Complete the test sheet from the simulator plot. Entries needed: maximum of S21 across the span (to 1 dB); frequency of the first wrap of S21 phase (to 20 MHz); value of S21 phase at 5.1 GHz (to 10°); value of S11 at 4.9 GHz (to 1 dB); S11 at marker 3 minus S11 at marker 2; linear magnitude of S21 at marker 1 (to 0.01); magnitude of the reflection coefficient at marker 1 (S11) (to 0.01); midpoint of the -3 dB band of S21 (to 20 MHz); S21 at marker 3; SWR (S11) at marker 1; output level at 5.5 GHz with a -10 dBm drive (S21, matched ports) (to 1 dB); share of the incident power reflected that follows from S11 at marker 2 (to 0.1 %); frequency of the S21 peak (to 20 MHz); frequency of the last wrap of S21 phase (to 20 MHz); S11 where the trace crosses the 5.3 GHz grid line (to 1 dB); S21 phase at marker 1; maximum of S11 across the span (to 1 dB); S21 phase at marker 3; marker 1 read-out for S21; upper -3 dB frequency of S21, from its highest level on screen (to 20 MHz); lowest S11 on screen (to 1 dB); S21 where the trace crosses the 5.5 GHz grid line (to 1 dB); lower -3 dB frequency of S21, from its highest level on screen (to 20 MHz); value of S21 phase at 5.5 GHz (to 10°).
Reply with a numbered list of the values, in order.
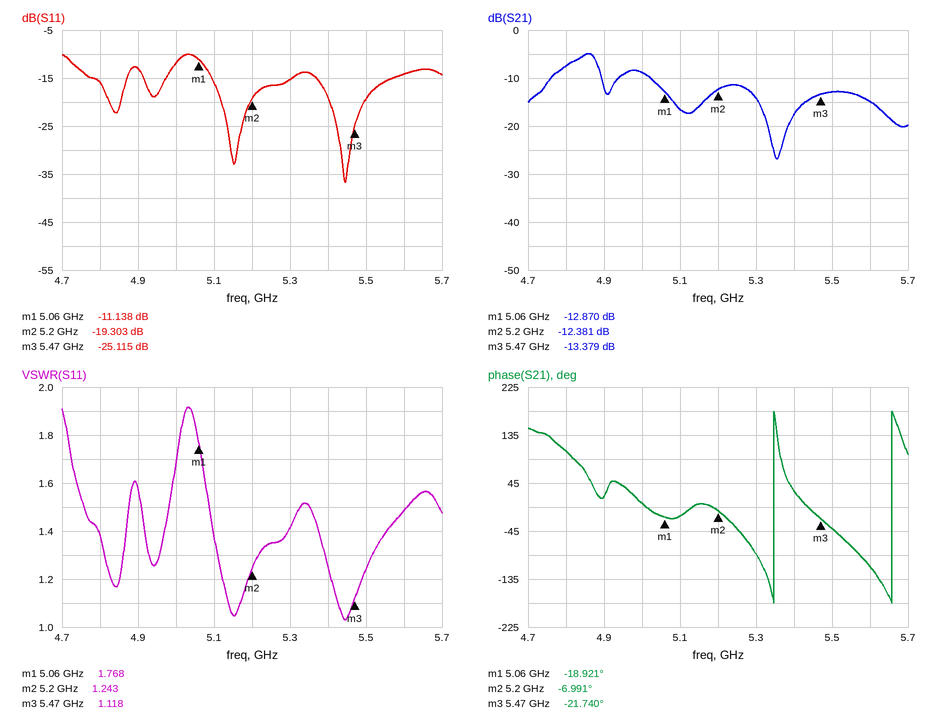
1. -5 dB
2. 5.34 GHz
3. -20°
4. -13 dB
5. -5.812 dB
6. 0.23
7. 0.28
8. 4.84 GHz
9. -13.379 dB
10. 1.768
11. -23 dBm
12. 1.2 %
13. 4.86 GHz
14. 5.66 GHz
15. -15 dB
16. -18.921°
17. -10 dB
18. -21.740°
19. -12.870 dB
20. 4.88 GHz
21. -37 dB
22. -13 dB
23. 4.80 GHz
24. -40°
